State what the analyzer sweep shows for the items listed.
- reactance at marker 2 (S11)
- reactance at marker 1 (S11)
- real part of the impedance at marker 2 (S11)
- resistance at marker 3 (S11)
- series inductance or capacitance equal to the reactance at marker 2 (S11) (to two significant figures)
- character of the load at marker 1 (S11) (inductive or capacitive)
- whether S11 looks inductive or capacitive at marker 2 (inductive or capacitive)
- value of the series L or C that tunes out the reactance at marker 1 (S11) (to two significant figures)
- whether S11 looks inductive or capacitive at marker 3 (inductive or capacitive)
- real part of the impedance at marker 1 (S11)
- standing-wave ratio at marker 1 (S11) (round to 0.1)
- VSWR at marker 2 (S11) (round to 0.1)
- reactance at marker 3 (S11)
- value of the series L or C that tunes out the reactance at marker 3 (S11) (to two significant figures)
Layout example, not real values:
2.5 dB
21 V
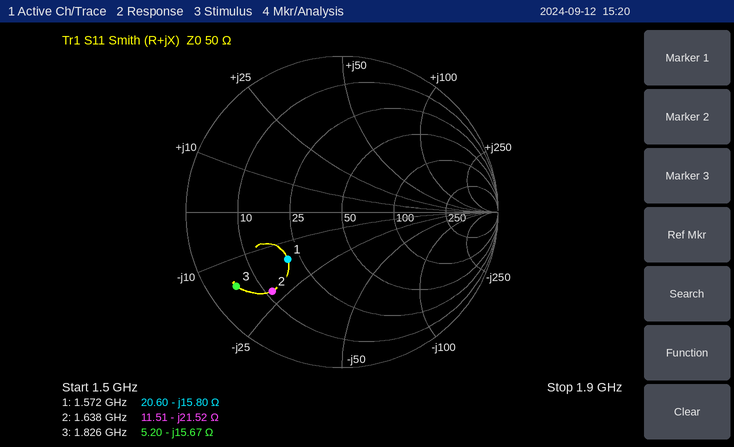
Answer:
-21.52 Ω
-15.80 Ω
11.51 Ω
5.20 Ω
4.5 pF
capacitive
capacitive
1.6 nH
capacitive
20.60 Ω
2.7
5.2
-15.67 Ω
1.4 nH
